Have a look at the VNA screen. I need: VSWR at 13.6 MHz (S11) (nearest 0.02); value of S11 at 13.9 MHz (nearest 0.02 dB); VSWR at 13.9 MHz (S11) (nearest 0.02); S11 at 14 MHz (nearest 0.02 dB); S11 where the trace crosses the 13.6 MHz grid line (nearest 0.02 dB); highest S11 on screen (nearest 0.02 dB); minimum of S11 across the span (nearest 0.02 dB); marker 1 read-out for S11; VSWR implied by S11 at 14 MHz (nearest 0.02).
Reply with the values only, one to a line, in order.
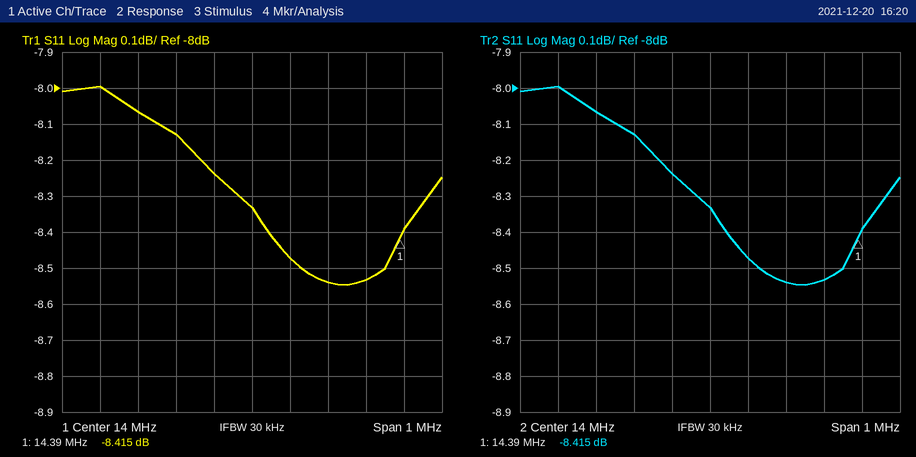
2.32
-8.24 dB
2.26
-8.34 dB
-8.00 dB
-8.00 dB
-8.54 dB
-8.415 dB
2.24
